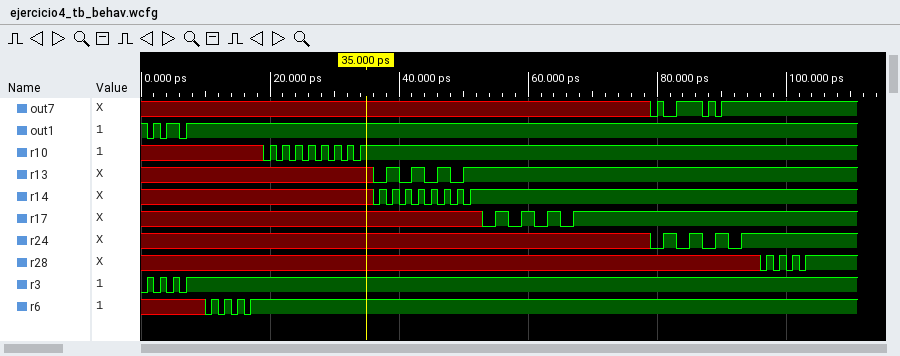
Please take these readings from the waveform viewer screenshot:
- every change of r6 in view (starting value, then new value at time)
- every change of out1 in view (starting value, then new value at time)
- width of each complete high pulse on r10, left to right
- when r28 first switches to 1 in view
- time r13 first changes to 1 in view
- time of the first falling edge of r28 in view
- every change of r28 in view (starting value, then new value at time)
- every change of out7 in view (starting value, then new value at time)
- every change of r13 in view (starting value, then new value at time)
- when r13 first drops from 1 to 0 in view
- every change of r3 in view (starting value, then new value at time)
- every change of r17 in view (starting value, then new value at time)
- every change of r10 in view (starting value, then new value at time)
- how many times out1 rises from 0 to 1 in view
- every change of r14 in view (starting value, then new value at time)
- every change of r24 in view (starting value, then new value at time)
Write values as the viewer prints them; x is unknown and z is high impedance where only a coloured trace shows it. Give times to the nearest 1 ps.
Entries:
x, 0 at 10 ps, 1 at 11 ps, 0 at 12 ps, 1 at 13 ps, 0 at 14 ps, 1 at 15 ps, 0 at 16 ps, 1 at 17 ps
1, 0 at 1 ps, 1 at 2 ps, 0 at 3 ps, 1 at 4 ps, 0 at 6 ps, 1 at 7 ps
1 ps, 1 ps, 1 ps, 1 ps, 1 ps, 1 ps, 1 ps
97 ps
38 ps
98 ps
x, 0 at 96 ps, 1 at 97 ps, 0 at 98 ps, 1 at 99 ps, 0 at 100 ps, 1 at 101 ps, 0 at 102 ps, 1 at 103 ps
x, 0 at 79 ps, 1 at 80 ps, 0 at 81 ps, 1 at 83 ps, 0 at 87 ps, 1 at 88 ps, 0 at 89 ps, 1 at 90 ps
x, 0 at 36 ps, 1 at 38 ps, 0 at 40 ps, 1 at 42 ps, 0 at 44 ps, 1 at 46 ps, 0 at 48 ps, 1 at 50 ps
40 ps
0, 1 at 1 ps, 0 at 2 ps, 1 at 3 ps, 0 at 4 ps, 1 at 5 ps, 0 at 6 ps, 1 at 7 ps
x, 0 at 53 ps, 1 at 55 ps, 0 at 57 ps, 1 at 59 ps, 0 at 61 ps, 1 at 63 ps, 0 at 65 ps, 1 at 67 ps
x, 0 at 19 ps, 1 at 20 ps, 0 at 21 ps, 1 at 22 ps, 0 at 23 ps, 1 at 24 ps, 0 at 25 ps, 1 at 26 ps, 0 at 27 ps, 1 at 28 ps, 0 at 29 ps, 1 at 30 ps, 0 at 31 ps, 1 at 32 ps, 0 at 33 ps, 1 at 34 ps
3
x, 0 at 36 ps, 1 at 37 ps, 0 at 38 ps, 1 at 39 ps, 0 at 40 ps, 1 at 41 ps, 0 at 42 ps, 1 at 43 ps, 0 at 44 ps, 1 at 45 ps, 0 at 46 ps, 1 at 47 ps, 0 at 48 ps, 1 at 49 ps, 0 at 50 ps, 1 at 51 ps
x, 0 at 79 ps, 1 at 81 ps, 0 at 83 ps, 1 at 85 ps, 0 at 87 ps, 1 at 89 ps, 0 at 91 ps, 1 at 93 ps
